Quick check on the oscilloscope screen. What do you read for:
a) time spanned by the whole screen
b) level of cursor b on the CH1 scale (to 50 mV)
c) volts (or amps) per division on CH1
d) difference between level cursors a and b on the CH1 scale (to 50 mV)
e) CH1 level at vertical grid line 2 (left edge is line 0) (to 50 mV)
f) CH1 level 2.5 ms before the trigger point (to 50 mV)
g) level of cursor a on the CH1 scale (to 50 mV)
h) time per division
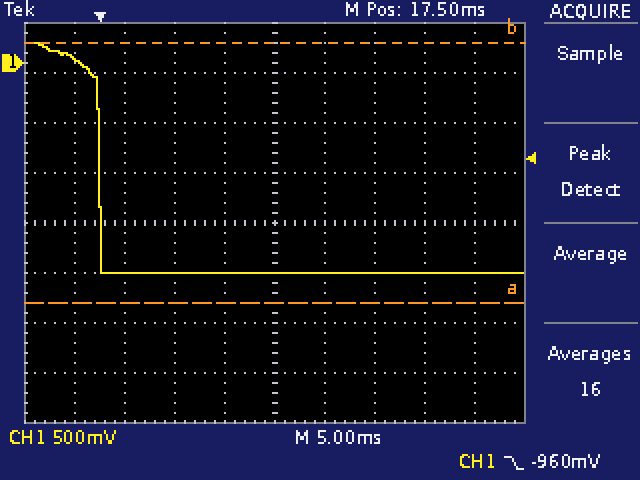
50 ms
200 mV
500 mV
2.60 V
-2.10 V
50 mV
-2.40 V
5 ms
